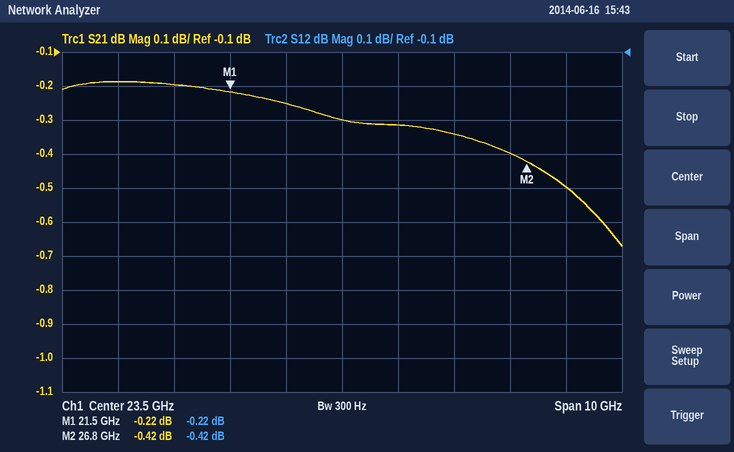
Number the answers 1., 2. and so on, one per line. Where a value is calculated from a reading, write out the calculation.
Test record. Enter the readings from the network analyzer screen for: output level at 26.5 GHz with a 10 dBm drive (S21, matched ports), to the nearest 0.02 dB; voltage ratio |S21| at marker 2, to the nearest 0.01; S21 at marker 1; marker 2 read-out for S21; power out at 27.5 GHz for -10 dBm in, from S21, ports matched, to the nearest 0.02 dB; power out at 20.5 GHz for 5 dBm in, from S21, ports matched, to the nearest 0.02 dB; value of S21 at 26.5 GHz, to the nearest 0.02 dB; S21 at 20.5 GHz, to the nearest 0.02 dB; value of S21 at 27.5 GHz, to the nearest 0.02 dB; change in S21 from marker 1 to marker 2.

1. 10 dBm + (-0.40 dB) = 9.60 dBm
2. 10^(-0.42/20) ≈ 0.95
3. -0.22 dB
4. -0.42 dB
5. -10 dBm + (-0.50 dB) = -10.50 dBm
6. 5 dBm + (-0.20 dB) = 4.80 dBm
7. -0.40 dB
8. -0.20 dB
9. -0.50 dB
10. -0.42 − (-0.22) = -0.20 dB
